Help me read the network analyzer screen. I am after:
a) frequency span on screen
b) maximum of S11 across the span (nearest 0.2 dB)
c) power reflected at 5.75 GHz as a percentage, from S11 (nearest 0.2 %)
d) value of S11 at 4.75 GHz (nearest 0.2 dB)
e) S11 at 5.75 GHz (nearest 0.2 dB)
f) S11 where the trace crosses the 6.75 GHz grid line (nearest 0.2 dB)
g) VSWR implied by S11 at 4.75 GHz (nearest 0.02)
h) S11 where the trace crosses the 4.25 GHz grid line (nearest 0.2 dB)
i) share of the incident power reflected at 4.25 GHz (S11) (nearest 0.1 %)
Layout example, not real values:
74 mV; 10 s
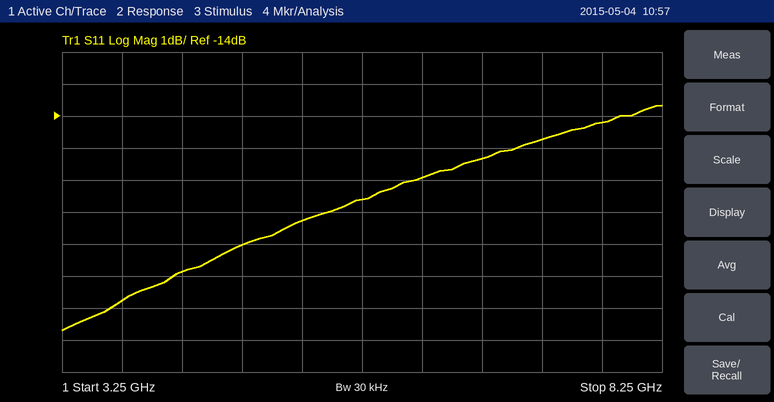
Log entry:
5 GHz; -13.6 dB; 2.2 %; -18.0 dB; -16.6 dB; -15.4 dB; 1.28; -18.8 dB; 1.3 %
